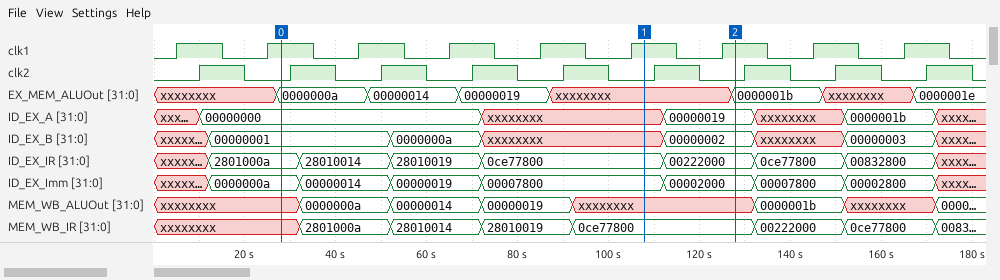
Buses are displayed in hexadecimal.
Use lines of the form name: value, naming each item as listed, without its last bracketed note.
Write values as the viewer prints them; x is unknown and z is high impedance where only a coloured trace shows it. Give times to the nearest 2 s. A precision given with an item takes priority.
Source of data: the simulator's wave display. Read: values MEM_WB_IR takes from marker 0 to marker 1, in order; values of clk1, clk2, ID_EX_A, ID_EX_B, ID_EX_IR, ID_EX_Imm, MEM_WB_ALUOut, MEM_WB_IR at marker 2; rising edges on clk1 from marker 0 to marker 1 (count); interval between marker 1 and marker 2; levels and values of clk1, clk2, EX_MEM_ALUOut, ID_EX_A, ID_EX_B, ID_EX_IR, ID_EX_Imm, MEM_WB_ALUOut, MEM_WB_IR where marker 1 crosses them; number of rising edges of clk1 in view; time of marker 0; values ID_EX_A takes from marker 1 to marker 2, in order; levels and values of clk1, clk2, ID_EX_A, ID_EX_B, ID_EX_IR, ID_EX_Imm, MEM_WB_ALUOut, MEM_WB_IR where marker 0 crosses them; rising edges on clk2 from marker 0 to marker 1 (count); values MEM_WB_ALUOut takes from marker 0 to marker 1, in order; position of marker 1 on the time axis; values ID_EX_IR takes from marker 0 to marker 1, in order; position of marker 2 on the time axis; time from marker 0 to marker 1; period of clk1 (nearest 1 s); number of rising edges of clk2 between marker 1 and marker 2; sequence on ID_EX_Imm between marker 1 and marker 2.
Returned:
values MEM_WB_IR takes from marker 0 to marker 1, in order: xxxxxxxx, 2801000a, 28010014, 28010019, 0ce77800
values of clk1, clk2, ID_EX_A, ID_EX_B, ID_EX_IR, ID_EX_Imm, MEM_WB_ALUOut, MEM_WB_IR at marker 2: clk1=1, clk2=0, ID_EX_A=00000019, ID_EX_B=00000002, ID_EX_IR=00222000, ID_EX_Imm=00002000, MEM_WB_ALUOut=xxxxxxxx, MEM_WB_IR=0ce77800
rising edges on clk1 from marker 0 to marker 1: 4
interval between marker 1 and marker 2: 20 s
levels and values of clk1, clk2, EX_MEM_ALUOut, ID_EX_A, ID_EX_B, ID_EX_IR, ID_EX_Imm, MEM_WB_ALUOut, MEM_WB_IR where marker 1 crosses them: clk1=1, clk2=0, EX_MEM_ALUOut=xxxxxxxx, ID_EX_A=xxxxxxxx, ID_EX_B=xxxxxxxx, ID_EX_IR=0ce77800, ID_EX_Imm=00007800, MEM_WB_ALUOut=xxxxxxxx, MEM_WB_IR=0ce77800
number of rising edges of clk1 in view: 9
time of marker 0: 28 s
values ID_EX_A takes from marker 1 to marker 2, in order: xxxxxxxx, 00000019
levels and values of clk1, clk2, ID_EX_A, ID_EX_B, ID_EX_IR, ID_EX_Imm, MEM_WB_ALUOut, MEM_WB_IR where marker 0 crosses them: clk1=1, clk2=0, ID_EX_A=00000000, ID_EX_B=00000001, ID_EX_IR=2801000a, ID_EX_Imm=0000000a, MEM_WB_ALUOut=xxxxxxxx, MEM_WB_IR=xxxxxxxx
rising edges on clk2 from marker 0 to marker 1: 4
values MEM_WB_ALUOut takes from marker 0 to marker 1, in order: xxxxxxxx, 0000000a, 00000014, 00000019, xxxxxxxx
position of marker 1 on the time axis: 108 s
values ID_EX_IR takes from marker 0 to marker 1, in order: 2801000a, 28010014, 28010019, 0ce77800
position of marker 2 on the time axis: 128 s
time from marker 0 to marker 1: 80 s
period of clk1: 20 s
number of rising edges of clk2 between marker 1 and marker 2: 1
sequence on ID_EX_Imm between marker 1 and marker 2: 00007800, 00002000
